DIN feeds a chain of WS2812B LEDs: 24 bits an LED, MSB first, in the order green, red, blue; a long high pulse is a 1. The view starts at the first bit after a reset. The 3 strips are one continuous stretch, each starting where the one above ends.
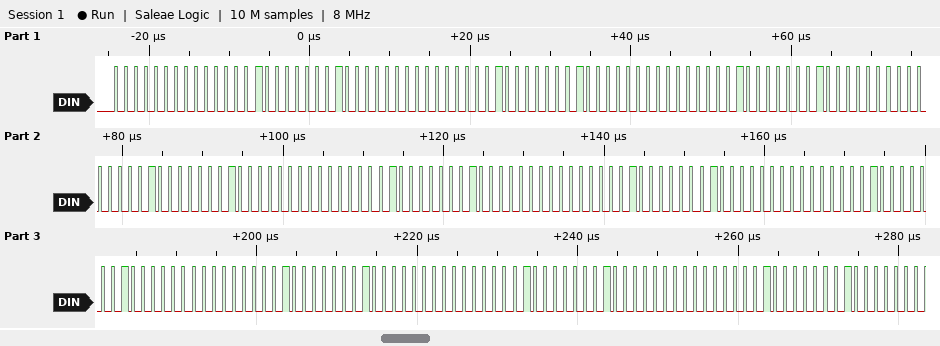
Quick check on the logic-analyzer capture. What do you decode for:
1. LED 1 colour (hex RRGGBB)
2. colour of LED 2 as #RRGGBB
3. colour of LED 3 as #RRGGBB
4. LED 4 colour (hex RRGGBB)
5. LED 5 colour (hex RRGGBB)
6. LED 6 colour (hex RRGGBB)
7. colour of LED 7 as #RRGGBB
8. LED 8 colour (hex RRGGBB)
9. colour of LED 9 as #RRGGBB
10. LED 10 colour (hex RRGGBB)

#020002
#020002
#020002
#020002
#020002
#020002
#020002
#020002
#020002
#020002
